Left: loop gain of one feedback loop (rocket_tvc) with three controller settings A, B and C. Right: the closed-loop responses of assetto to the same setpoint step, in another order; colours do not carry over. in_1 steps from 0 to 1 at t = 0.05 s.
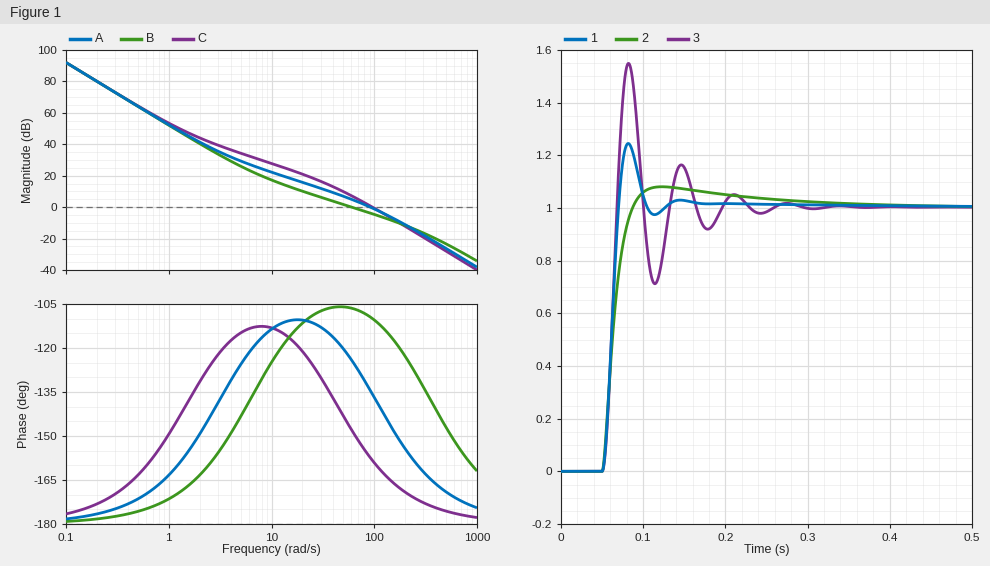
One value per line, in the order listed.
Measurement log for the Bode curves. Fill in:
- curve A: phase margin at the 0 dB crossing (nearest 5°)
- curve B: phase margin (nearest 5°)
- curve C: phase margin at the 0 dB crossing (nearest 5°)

45°
75°
20°
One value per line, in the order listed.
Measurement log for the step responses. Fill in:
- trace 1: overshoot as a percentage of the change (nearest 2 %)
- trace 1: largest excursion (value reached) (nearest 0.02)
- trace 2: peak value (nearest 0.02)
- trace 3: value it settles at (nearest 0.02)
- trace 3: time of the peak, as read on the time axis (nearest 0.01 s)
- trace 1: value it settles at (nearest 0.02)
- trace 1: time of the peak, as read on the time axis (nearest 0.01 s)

24 %
1.24
1.08
1.00
0.08 s
1.00
0.08 s
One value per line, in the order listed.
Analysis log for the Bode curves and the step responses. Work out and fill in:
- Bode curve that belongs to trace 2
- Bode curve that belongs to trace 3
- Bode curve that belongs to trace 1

B
C
A
